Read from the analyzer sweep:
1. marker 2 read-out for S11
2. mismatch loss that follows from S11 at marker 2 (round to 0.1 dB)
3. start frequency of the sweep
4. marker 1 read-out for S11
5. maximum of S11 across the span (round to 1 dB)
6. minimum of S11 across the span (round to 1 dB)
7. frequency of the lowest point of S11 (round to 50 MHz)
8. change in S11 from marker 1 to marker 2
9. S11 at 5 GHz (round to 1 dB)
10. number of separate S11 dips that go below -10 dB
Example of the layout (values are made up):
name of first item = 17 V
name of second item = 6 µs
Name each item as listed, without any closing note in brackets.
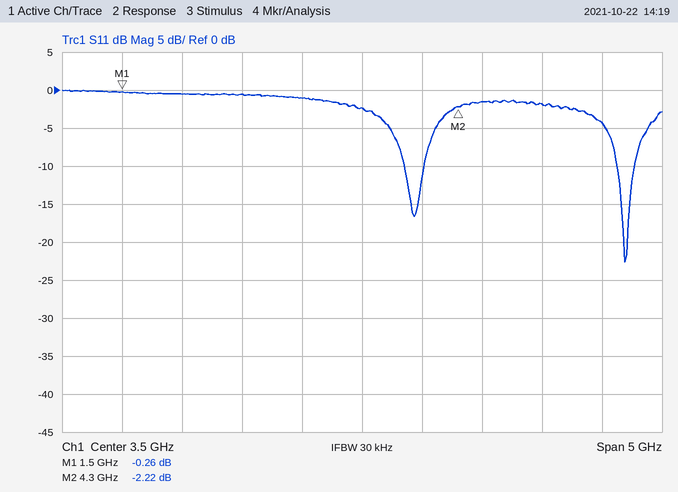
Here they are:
marker 2 read-out for S11 = -2.22 dB
mismatch loss that follows from S11 at marker 2 = 4.0 dB
start frequency of the sweep = 1 GHz
marker 1 read-out for S11 = -0.26 dB
maximum of S11 across the span = 0 dB
minimum of S11 across the span = -23 dB
frequency of the lowest point of S11 = 5.70 GHz
change in S11 from marker 1 to marker 2 = -1.96 dB
S11 at 5 GHz = -2 dB
number of separate S11 dips that go below -10 dB = 2
